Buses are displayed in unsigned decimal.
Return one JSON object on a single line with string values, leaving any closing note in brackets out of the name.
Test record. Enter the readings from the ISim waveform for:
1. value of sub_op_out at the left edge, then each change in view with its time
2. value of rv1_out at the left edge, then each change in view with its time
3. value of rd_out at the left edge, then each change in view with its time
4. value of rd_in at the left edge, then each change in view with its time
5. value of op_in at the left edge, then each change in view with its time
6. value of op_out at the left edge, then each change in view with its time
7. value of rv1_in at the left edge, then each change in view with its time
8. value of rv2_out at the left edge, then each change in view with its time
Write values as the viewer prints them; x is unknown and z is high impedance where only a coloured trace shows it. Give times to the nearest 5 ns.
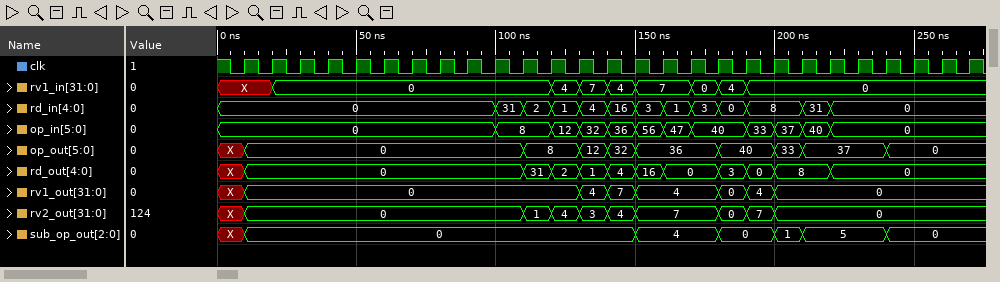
{"value of sub_op_out at the left edge, then each change in view with its time": "X, 0 at 10 ns, 4 at 150 ns, 0 at 180 ns, 1 at 200 ns, 5 at 210 ns, 0 at 240 ns", "value of rv1_out at the left edge, then each change in view with its time": "X, 0 at 10 ns, 4 at 130 ns, 7 at 140 ns, 4 at 150 ns, 0 at 180 ns, 4 at 190 ns, 0 at 200 ns", "value of rd_out at the left edge, then each change in view with its time": "X, 0 at 10 ns, 31 at 110 ns, 2 at 120 ns, 1 at 130 ns, 4 at 140 ns, 16 at 150 ns, 0 at 160 ns, 3 at 180 ns, 0 at 190 ns, 8 at 200 ns, 0 at 220 ns", "value of rd_in at the left edge, then each change in view with its time": "0, 31 at 100 ns, 2 at 110 ns, 1 at 120 ns, 4 at 130 ns, 16 at 140 ns, 3 at 150 ns, 1 at 160 ns, 3 at 170 ns, 0 at 180 ns, 8 at 190 ns, 31 at 210 ns, 0 at 220 ns", "value of op_in at the left edge, then each change in view with its time": "0, 8 at 100 ns, 12 at 120 ns, 32 at 130 ns, 36 at 140 ns, 56 at 150 ns, 47 at 160 ns, 40 at 170 ns, 33 at 190 ns, 37 at 200 ns, 40 at 210 ns, 0 at 220 ns", "value of op_out at the left edge, then each change in view with its time": "X, 0 at 10 ns, 8 at 110 ns, 12 at 130 ns, 32 at 140 ns, 36 at 150 ns, 40 at 180 ns, 33 at 200 ns, 37 at 210 ns, 0 at 240 ns", "value of rv1_in at the left edge, then each change in view with its time": "X, 0 at 20 ns, 4 at 120 ns, 7 at 130 ns, 4 at 140 ns, 7 at 150 ns, 0 at 170 ns, 4 at 180 ns, 0 at 190 ns", "value of rv2_out at the left edge, then each change in view with its time": "X, 0 at 10 ns, 1 at 110 ns, 4 at 120 ns, 3 at 130 ns, 4 at 140 ns, 7 at 150 ns, 0 at 180 ns, 7 at 190 ns, 0 at 200 ns"}
